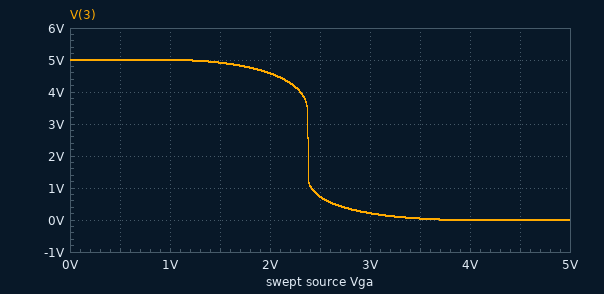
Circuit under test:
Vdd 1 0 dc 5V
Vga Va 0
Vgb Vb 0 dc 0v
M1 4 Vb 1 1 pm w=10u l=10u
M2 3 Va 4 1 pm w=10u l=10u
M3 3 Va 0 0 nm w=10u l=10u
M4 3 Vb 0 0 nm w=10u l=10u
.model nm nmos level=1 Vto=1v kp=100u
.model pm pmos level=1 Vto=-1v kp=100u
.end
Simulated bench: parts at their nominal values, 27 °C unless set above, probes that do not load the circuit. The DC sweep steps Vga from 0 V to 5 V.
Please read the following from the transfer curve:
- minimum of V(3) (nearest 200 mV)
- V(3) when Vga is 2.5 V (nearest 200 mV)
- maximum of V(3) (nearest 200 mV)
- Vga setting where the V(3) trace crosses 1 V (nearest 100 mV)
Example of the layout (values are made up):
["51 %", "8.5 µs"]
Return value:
["0 V", "800 mV", "5.0 V", "2.4 V"]
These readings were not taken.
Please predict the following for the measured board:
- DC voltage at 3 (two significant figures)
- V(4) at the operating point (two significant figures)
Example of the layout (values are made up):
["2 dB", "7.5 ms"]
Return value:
["5.0 V", "5.0 V"]
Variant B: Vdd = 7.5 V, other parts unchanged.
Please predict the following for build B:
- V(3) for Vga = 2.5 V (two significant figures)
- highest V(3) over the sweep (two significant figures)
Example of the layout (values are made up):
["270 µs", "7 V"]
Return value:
["7.0 V", "7.5 V"]
